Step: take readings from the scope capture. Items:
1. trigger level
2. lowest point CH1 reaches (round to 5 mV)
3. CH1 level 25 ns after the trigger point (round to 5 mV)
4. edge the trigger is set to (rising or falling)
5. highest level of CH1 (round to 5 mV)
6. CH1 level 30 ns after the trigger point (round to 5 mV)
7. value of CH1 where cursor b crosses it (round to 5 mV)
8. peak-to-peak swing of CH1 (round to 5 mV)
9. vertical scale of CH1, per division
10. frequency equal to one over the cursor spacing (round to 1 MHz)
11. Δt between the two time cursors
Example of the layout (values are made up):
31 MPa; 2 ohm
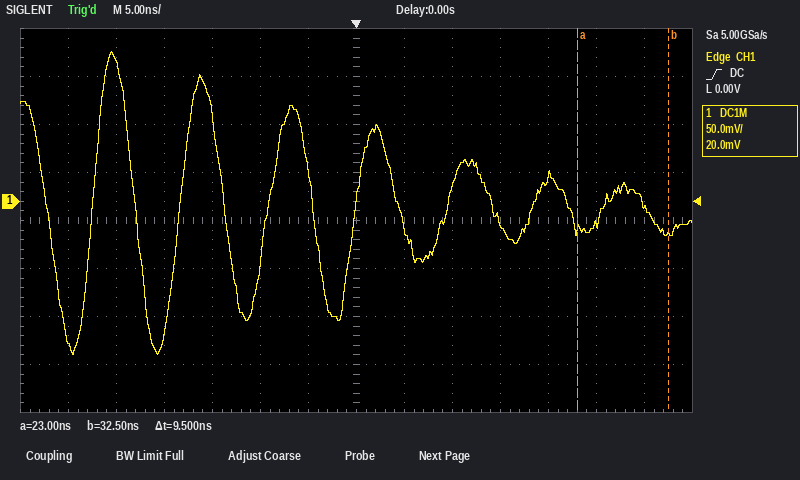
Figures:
0.00 V; -160 mV; -25 mV; rising; 155 mV; -5 mV; -35 mV; 315 mV; 50 mV; 105 MHz; 9.5 ns
